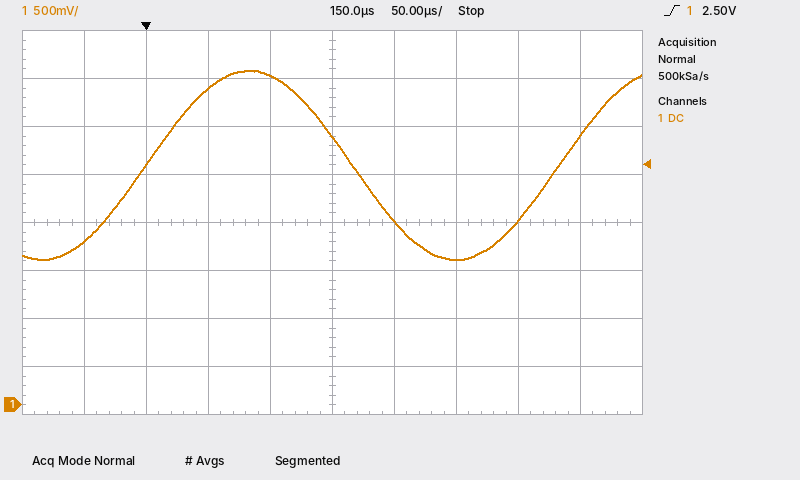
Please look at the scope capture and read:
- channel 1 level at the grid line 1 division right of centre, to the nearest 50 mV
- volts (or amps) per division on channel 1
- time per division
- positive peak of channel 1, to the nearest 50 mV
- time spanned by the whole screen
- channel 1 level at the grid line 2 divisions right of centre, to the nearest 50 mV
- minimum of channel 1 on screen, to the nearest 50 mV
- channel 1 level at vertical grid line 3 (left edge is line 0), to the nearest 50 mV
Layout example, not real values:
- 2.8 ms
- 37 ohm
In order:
- 1.90 V
- 500 mV
- 50 µs
- 3.50 V
- 500 µs
- 1.50 V
- 1.50 V
- 3.30 V
